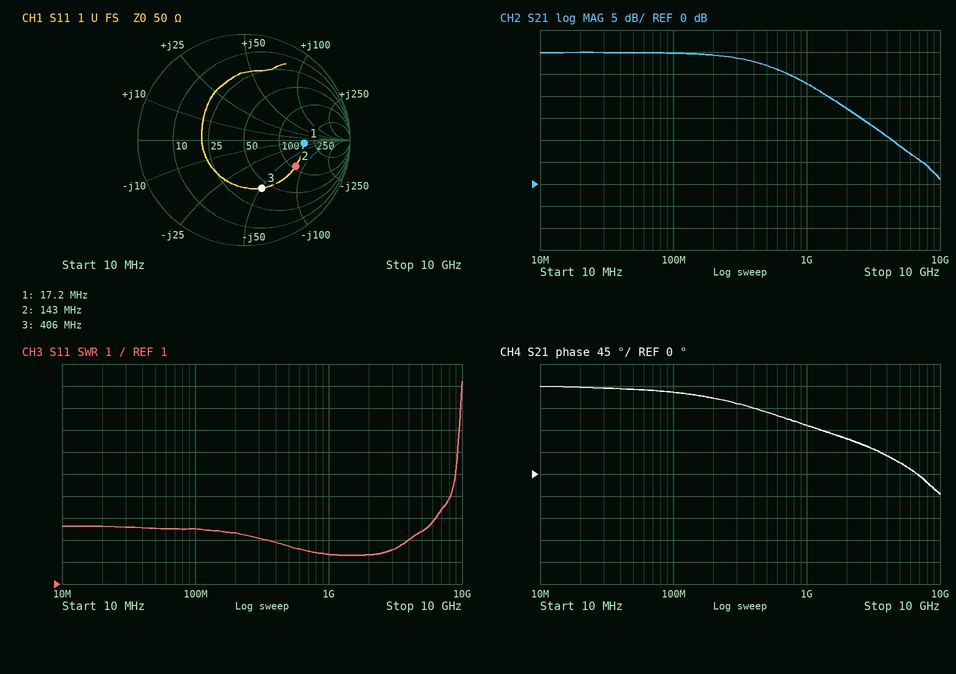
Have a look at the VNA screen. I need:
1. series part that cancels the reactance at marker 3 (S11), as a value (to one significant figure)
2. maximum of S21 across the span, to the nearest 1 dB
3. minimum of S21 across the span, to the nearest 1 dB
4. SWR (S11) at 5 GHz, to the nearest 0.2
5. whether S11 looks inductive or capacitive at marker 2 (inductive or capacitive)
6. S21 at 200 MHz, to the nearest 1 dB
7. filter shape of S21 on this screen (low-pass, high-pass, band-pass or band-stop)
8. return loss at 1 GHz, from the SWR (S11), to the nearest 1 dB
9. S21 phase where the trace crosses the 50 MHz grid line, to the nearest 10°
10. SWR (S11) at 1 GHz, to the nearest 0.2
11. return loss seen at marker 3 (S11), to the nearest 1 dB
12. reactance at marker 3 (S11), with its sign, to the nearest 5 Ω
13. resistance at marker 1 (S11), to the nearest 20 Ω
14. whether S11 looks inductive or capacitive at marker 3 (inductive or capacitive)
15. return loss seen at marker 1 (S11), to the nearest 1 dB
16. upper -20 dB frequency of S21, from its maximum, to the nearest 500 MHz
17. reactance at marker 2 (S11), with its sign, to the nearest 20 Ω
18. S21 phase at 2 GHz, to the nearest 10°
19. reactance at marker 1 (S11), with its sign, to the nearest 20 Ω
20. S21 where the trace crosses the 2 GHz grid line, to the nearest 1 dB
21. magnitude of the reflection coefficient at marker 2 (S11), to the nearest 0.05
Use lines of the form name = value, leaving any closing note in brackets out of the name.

series part that cancels the reactance at marker 3 (S11), as a value = 20 nH
maximum of S21 across the span, to the nearest 1 dB = 30 dB
minimum of S21 across the span, to the nearest 1 dB = 1 dB
SWR (S11) at 5 GHz, to the nearest 0.2 = 3.4
whether S11 looks inductive or capacitive at marker 2 = capacitive
S21 at 200 MHz, to the nearest 1 dB = 29 dB
filter shape of S21 on this screen = low-pass
return loss at 1 GHz, from the SWR (S11), to the nearest 1 dB = 8 dB
S21 phase where the trace crosses the 50 MHz grid line, to the nearest 10° = 170°
SWR (S11) at 1 GHz, to the nearest 0.2 = 2.4
return loss seen at marker 3 (S11), to the nearest 1 dB = 6 dB
reactance at marker 3 (S11), with its sign, to the nearest 5 Ω = -50 Ω
resistance at marker 1 (S11), to the nearest 20 Ω = 180 Ω
whether S11 looks inductive or capacitive at marker 3 = capacitive
return loss seen at marker 1 (S11), to the nearest 1 dB = 5 dB
upper -20 dB frequency of S21, from its maximum, to the nearest 500 MHz = 4.5 GHz
reactance at marker 2 (S11), with its sign, to the nearest 20 Ω = -80 Ω
S21 phase at 2 GHz, to the nearest 10° = 70°
reactance at marker 1 (S11), with its sign, to the nearest 20 Ω = -20 Ω
S21 where the trace crosses the 2 GHz grid line, to the nearest 1 dB = 17 dB
magnitude of the reflection coefficient at marker 2 (S11), to the nearest 0.05 = 0.55
